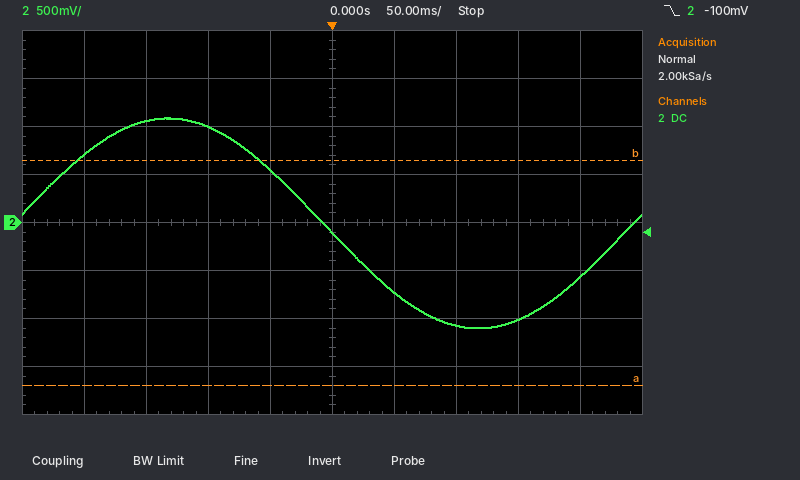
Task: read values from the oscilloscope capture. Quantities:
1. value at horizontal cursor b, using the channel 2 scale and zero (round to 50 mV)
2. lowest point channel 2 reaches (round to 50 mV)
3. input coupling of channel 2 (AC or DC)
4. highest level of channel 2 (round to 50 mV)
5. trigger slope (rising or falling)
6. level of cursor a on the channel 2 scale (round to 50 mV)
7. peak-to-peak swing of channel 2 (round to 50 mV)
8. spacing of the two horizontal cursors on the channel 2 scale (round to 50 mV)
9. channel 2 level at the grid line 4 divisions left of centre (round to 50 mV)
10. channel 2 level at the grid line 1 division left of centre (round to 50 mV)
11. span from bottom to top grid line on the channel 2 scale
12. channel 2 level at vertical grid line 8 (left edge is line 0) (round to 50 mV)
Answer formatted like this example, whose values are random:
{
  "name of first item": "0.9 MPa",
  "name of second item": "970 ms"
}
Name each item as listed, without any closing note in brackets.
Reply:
{
  "value at horizontal cursor b, using the channel 2 scale and zero": "650 mV",
  "lowest point channel 2 reaches": "-1.10 V",
  "input coupling of channel 2": "DC",
  "highest level of channel 2": "1.10 V",
  "trigger slope": "falling",
  "level of cursor a on the channel 2 scale": "-1.70 V",
  "peak-to-peak swing of channel 2": "2.20 V",
  "spacing of the two horizontal cursors on the channel 2 scale": "2.35 V",
  "channel 2 level at the grid line 4 divisions left of centre": "700 mV",
  "channel 2 level at the grid line 1 division left of centre": "550 mV",
  "span from bottom to top grid line on the channel 2 scale": "4 V",
  "channel 2 level at vertical grid line 8 (left edge is line 0)": "-1.00 V"
}
